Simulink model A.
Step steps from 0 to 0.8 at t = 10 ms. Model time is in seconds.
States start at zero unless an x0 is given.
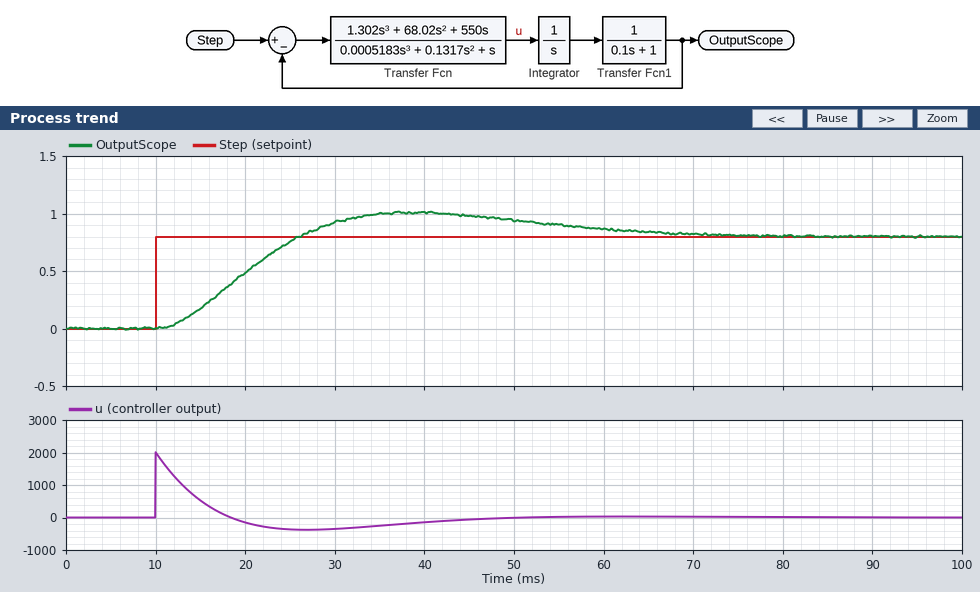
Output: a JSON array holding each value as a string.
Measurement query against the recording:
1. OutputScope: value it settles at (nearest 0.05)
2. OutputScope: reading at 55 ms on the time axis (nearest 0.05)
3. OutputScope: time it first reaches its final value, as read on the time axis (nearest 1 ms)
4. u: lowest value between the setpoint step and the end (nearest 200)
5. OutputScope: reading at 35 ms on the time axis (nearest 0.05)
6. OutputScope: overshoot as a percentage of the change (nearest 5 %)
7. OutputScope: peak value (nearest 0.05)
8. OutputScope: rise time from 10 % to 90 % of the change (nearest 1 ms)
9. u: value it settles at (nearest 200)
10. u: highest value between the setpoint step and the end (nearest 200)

["0.80", "0.90", "26 ms", "-400", "1.00", "25 %", "1.00", "11 ms", "0", "2000"]
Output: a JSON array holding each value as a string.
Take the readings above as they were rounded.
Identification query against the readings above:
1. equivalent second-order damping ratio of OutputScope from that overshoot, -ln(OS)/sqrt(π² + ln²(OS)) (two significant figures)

["0.40"]
